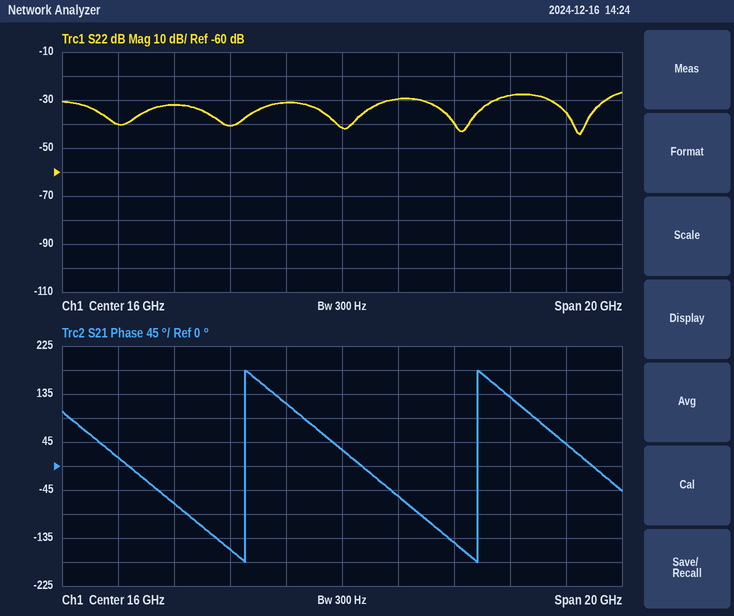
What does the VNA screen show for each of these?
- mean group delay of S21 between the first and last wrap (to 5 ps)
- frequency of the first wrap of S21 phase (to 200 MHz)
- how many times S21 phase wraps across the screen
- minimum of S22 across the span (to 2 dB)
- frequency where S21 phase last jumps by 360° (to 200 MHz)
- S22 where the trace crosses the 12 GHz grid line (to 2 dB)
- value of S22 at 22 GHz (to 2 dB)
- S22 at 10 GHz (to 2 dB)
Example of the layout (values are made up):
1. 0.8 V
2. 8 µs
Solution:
1. 120 ps
2. 12.6 GHz
3. 2
4. -44 dB
5. 20.8 GHz
6. -40 dB
7. -28 dB
8. -32 dB
